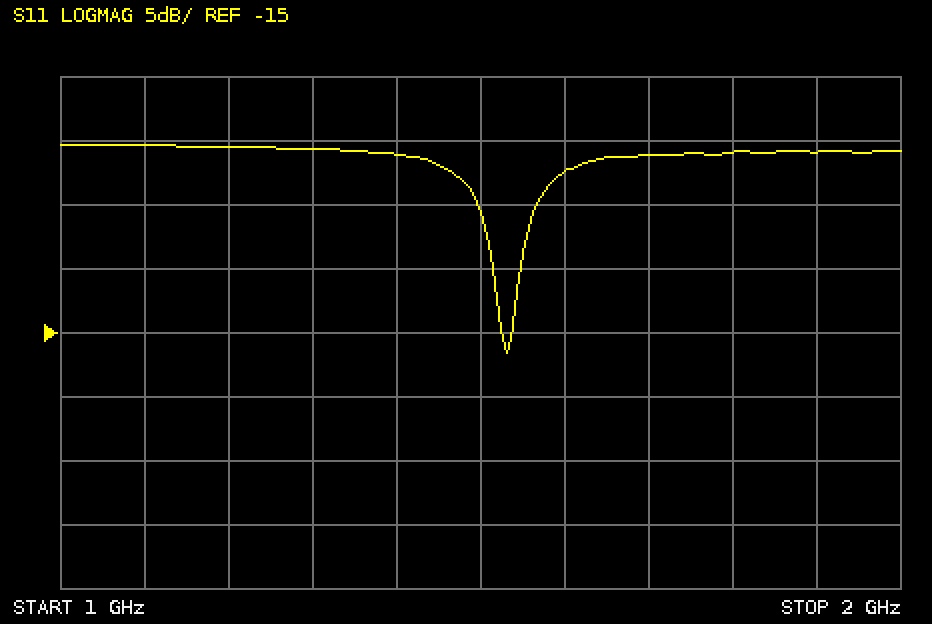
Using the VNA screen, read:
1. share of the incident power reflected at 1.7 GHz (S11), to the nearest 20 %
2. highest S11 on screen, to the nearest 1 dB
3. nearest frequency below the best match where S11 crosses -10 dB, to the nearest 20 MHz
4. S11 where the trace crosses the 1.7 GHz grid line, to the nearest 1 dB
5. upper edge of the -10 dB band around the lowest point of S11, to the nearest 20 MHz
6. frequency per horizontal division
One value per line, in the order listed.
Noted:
80 %
0 dB
1.52 GHz
-1 dB
1.54 GHz
100 MHz
